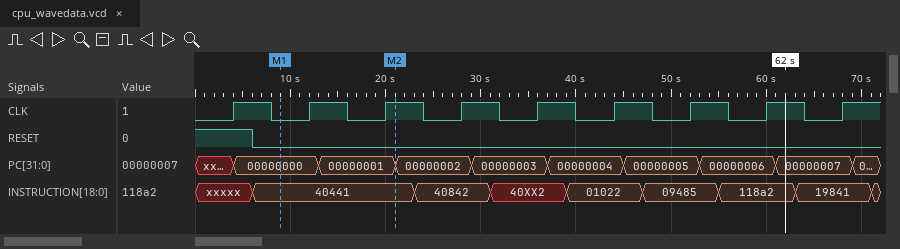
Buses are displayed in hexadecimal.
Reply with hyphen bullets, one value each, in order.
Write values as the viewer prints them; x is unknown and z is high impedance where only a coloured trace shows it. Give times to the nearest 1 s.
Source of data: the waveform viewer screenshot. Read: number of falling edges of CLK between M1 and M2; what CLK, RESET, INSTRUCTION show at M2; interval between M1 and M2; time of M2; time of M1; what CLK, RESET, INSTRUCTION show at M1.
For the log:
- 1
- CLK=1, RESET=0, INSTRUCTION=40441
- 12 s
- 21 s
- 9 s
- CLK=0, RESET=0, INSTRUCTION=40441
